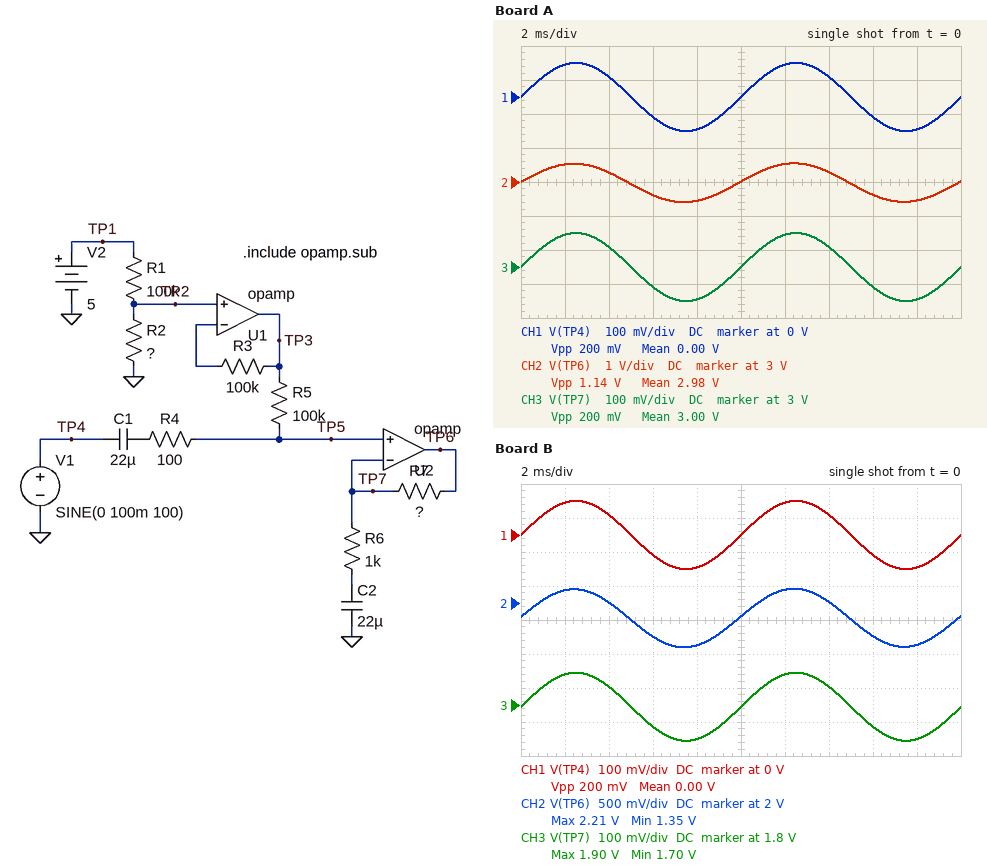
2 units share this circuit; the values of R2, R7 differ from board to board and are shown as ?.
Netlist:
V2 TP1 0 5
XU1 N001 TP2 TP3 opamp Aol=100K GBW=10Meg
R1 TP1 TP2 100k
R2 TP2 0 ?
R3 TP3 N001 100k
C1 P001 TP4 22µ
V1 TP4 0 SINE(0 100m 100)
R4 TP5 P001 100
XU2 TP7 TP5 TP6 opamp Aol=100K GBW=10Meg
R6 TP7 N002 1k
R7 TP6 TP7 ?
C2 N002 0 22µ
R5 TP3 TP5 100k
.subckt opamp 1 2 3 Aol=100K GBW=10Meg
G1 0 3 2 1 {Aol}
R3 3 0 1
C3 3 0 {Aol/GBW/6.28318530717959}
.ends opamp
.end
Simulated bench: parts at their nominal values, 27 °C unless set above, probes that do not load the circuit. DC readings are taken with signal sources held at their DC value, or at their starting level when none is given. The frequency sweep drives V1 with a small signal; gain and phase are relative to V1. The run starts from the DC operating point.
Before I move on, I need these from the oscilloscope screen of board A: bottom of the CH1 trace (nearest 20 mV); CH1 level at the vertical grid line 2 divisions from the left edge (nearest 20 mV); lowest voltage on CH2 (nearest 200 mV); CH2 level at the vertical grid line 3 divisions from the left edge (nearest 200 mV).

-100 mV
60 mV
2.4 V
2.6 V
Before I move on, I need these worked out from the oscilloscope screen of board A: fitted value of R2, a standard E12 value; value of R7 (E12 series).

150 kΩ
4.7 kΩ
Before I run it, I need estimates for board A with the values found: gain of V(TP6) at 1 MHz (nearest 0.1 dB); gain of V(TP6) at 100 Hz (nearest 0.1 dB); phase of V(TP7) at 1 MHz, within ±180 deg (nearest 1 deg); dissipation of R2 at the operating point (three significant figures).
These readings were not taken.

13.9 dB
15.1 dB
-30 deg
60.0 µW
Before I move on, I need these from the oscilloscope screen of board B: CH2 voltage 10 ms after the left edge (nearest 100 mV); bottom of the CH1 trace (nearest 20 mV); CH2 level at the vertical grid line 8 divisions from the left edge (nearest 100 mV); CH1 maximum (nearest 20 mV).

1.8 V
-100 mV
1.5 V
100 mV
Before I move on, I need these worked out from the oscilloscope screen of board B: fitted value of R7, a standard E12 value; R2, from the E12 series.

3.3 kΩ
56 kΩ
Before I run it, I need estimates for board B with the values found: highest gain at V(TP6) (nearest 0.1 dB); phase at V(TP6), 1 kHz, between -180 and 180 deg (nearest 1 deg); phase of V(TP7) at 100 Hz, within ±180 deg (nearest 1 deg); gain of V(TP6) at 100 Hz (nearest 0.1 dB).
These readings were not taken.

12.7 dB
0 deg
0 deg
12.6 dB
